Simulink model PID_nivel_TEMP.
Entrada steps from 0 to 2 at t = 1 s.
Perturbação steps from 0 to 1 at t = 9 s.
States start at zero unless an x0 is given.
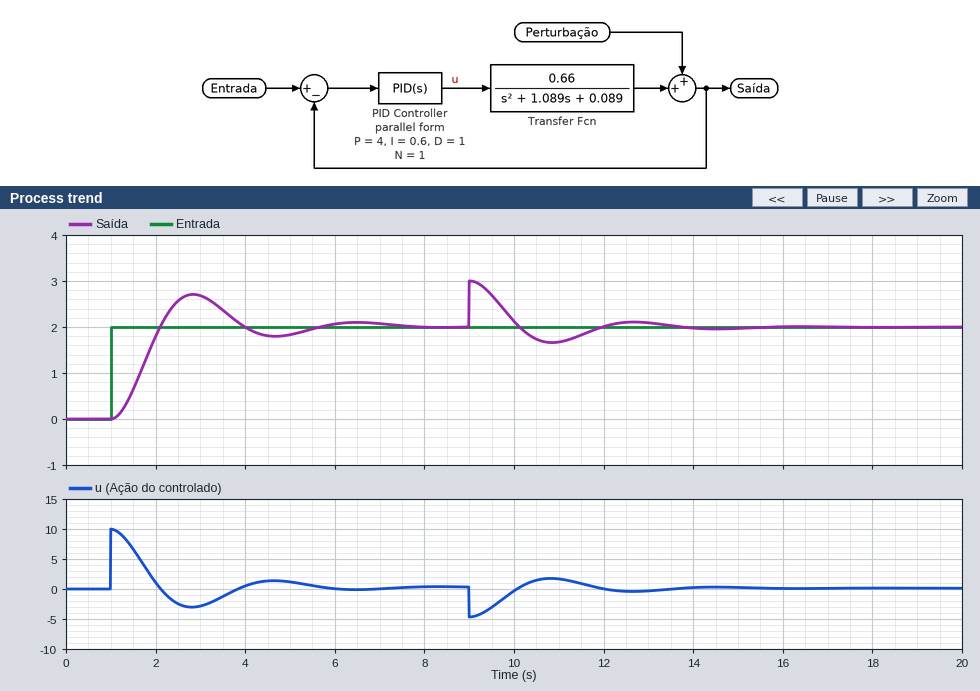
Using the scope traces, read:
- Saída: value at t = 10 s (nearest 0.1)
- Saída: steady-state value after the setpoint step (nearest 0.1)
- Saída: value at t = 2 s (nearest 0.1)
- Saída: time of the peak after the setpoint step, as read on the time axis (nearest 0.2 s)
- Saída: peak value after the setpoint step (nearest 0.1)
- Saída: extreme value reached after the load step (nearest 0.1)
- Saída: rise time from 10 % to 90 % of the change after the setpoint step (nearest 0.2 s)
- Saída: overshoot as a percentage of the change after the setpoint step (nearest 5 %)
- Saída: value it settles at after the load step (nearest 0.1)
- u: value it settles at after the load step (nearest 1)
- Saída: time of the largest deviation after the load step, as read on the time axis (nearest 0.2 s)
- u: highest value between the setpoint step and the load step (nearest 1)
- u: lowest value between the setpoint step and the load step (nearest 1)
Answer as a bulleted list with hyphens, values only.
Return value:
- 2.1
- 2.0
- 1.8
- 2.8 s
- 2.7
- 3.0
- 0.8 s
- 35 %
- 2.0
- 0
- 9.0 s
- 10
- -3
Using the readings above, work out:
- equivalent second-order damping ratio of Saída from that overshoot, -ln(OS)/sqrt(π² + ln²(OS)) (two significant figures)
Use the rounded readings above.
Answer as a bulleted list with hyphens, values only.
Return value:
- 0.32
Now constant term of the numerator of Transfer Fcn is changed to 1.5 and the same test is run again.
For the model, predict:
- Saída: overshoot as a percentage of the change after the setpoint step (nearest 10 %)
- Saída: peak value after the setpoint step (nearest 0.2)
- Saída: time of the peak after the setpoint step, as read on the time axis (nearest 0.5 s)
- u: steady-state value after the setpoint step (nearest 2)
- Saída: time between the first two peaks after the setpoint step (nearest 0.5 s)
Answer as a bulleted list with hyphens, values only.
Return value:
- 50 %
- 3.0
- 2.0 s
- 0
- 2.5 s
